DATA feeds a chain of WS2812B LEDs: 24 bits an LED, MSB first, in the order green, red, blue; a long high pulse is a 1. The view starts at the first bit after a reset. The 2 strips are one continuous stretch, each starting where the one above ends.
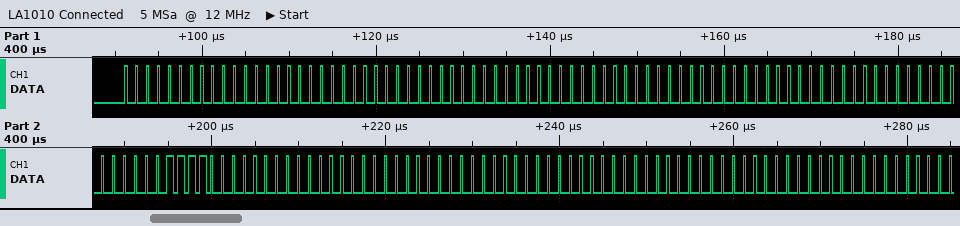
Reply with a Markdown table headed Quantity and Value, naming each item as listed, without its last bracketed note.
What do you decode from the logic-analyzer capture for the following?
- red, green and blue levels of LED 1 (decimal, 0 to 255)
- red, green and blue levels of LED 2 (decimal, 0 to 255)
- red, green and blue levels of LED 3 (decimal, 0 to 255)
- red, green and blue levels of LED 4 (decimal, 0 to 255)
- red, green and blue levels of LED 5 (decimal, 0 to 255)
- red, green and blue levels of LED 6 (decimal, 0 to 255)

| Quantity | Value |
|---|---|
| red, green and blue levels of LED 1 | 0, 0, 0 |
| red, green and blue levels of LED 2 | 0, 0, 0 |
| red, green and blue levels of LED 3 | 0, 0, 0 |
| red, green and blue levels of LED 4 | 30, 0, 0 |
| red, green and blue levels of LED 5 | 0, 0, 0 |
| red, green and blue levels of LED 6 | 0, 0, 0 |
